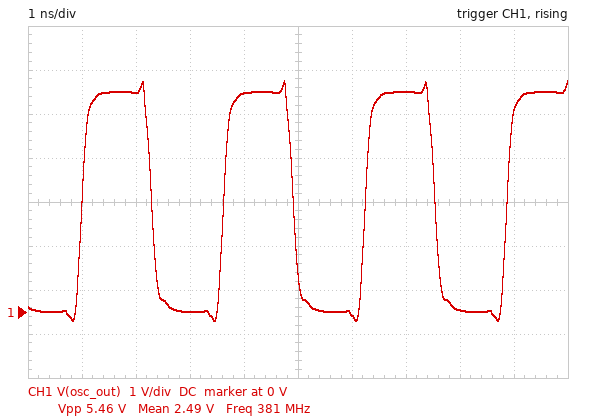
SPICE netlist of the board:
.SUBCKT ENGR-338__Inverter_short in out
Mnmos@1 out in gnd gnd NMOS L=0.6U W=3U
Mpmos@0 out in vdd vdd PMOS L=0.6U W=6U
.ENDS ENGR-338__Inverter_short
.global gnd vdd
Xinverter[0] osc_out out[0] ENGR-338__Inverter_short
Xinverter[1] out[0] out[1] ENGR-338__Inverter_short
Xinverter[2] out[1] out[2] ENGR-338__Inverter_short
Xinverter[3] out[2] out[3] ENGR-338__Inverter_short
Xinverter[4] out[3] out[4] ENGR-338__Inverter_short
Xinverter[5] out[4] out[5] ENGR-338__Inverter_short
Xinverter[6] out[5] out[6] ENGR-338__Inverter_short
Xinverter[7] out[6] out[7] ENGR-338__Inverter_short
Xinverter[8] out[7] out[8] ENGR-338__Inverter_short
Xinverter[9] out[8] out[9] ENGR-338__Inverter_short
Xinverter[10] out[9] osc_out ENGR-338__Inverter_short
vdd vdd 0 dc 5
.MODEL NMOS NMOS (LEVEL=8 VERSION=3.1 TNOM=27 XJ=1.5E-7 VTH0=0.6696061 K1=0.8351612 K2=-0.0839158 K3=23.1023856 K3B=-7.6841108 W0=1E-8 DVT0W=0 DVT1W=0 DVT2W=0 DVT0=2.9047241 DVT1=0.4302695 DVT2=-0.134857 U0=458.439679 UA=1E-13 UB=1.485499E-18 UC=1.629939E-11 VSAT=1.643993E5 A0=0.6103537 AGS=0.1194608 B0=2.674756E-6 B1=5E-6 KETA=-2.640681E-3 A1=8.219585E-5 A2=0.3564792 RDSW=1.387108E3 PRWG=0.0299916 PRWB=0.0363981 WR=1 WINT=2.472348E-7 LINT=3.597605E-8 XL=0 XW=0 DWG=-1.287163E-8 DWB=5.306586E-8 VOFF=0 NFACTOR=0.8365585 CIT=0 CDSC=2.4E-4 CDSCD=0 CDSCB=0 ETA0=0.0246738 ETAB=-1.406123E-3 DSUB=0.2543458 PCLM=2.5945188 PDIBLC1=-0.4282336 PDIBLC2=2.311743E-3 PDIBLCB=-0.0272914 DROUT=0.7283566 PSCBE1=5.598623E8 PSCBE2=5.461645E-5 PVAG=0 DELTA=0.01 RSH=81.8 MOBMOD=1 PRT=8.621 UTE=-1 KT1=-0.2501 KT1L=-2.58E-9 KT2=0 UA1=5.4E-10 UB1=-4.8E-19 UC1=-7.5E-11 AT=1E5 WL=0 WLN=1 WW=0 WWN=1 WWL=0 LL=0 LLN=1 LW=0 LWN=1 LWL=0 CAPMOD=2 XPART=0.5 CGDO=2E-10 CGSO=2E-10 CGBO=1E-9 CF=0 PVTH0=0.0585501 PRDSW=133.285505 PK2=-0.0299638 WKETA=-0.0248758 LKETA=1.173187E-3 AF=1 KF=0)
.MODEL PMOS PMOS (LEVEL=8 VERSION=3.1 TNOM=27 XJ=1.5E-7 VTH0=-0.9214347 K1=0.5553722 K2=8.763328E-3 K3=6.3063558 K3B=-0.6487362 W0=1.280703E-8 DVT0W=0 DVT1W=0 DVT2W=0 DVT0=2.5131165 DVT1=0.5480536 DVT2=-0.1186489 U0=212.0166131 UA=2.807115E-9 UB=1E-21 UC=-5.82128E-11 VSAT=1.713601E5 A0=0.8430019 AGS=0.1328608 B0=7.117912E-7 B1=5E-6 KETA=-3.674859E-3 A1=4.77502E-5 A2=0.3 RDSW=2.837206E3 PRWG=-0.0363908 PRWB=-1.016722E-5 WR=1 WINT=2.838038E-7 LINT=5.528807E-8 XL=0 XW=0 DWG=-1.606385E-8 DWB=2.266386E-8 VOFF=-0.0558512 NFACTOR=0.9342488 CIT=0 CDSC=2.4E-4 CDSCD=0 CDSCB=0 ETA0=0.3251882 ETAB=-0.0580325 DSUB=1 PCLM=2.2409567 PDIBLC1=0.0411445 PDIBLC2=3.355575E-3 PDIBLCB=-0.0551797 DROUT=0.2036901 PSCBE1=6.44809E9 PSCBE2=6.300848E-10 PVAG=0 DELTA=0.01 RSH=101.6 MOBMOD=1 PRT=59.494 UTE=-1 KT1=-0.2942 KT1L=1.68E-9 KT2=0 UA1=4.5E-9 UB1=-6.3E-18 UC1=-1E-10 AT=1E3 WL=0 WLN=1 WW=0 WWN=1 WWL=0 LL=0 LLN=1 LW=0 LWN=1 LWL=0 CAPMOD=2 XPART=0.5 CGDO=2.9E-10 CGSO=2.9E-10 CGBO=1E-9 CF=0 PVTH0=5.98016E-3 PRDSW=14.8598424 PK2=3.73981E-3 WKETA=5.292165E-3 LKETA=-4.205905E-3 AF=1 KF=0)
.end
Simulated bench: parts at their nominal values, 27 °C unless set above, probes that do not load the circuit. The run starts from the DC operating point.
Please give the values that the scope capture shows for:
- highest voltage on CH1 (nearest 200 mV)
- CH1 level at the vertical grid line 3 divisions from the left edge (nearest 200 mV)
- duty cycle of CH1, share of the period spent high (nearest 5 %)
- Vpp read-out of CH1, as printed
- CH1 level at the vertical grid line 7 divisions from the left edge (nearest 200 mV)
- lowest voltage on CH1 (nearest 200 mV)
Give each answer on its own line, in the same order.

5.2 V
0 V
50 %
5.46 V
5.0 V
-200 mV
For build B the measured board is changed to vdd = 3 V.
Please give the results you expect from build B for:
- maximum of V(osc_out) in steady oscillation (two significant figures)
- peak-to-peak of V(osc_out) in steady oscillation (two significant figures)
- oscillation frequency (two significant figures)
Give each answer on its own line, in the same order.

3.3 V
3.5 V
270 MHz
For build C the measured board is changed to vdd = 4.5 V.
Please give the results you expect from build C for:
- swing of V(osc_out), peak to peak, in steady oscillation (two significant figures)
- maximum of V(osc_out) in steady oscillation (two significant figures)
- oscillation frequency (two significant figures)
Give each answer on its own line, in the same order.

5.0 V
4.8 V
360 MHz
